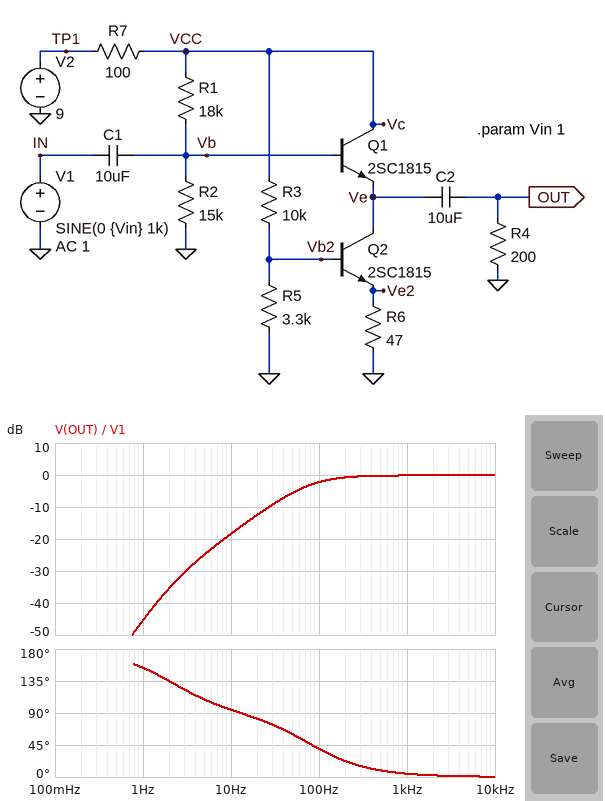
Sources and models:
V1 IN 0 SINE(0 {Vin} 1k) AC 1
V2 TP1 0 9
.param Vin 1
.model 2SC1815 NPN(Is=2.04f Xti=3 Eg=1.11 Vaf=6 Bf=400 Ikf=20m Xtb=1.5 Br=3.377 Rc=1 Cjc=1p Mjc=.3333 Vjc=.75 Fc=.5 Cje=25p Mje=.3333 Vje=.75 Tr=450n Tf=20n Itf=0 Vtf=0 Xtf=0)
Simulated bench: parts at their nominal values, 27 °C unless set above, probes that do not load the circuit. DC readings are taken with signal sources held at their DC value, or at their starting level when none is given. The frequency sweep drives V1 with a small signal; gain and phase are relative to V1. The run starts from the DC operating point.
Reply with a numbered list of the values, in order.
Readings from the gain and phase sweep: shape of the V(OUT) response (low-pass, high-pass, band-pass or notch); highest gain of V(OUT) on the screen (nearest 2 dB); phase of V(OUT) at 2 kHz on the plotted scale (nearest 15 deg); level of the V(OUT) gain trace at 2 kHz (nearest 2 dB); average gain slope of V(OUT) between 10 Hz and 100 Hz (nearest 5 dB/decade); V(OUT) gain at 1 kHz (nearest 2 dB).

1. high-pass
2. 0 dB
3. 0 deg
4. 0 dB
5. 15 dB/decade
6. 0 dB
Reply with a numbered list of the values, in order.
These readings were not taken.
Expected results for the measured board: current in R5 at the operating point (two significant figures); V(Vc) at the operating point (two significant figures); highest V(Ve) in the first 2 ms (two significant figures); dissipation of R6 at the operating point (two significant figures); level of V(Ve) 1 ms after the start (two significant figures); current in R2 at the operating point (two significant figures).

1. 490 µA
2. 7.2 V
3. 3.2 V
4. 14 mW
5. 2.2 V
6. 200 µA
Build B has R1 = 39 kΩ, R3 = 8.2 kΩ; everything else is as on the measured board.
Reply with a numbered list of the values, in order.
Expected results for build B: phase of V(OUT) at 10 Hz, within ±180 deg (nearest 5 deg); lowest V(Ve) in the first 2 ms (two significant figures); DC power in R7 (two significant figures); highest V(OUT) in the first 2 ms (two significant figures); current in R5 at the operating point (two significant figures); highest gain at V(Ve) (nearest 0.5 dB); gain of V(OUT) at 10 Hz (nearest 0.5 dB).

1. 100 deg
2. 240 mV
3. 30 mW
4. 910 mV
5. 480 µA
6. -0.5 dB
7. -19.0 dB
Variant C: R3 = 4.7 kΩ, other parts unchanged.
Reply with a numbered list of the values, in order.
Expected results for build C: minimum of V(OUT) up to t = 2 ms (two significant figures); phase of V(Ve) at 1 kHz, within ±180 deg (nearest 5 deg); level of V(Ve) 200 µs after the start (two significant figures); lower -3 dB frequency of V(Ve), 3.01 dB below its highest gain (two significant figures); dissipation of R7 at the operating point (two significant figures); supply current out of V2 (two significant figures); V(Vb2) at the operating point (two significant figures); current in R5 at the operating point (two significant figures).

1. -980 mV
2. 0 deg
3. 2.4 V
4. 4.4 Hz
5. 77 mW
6. 28 mA
7. 2.1 V
8. 630 µA
